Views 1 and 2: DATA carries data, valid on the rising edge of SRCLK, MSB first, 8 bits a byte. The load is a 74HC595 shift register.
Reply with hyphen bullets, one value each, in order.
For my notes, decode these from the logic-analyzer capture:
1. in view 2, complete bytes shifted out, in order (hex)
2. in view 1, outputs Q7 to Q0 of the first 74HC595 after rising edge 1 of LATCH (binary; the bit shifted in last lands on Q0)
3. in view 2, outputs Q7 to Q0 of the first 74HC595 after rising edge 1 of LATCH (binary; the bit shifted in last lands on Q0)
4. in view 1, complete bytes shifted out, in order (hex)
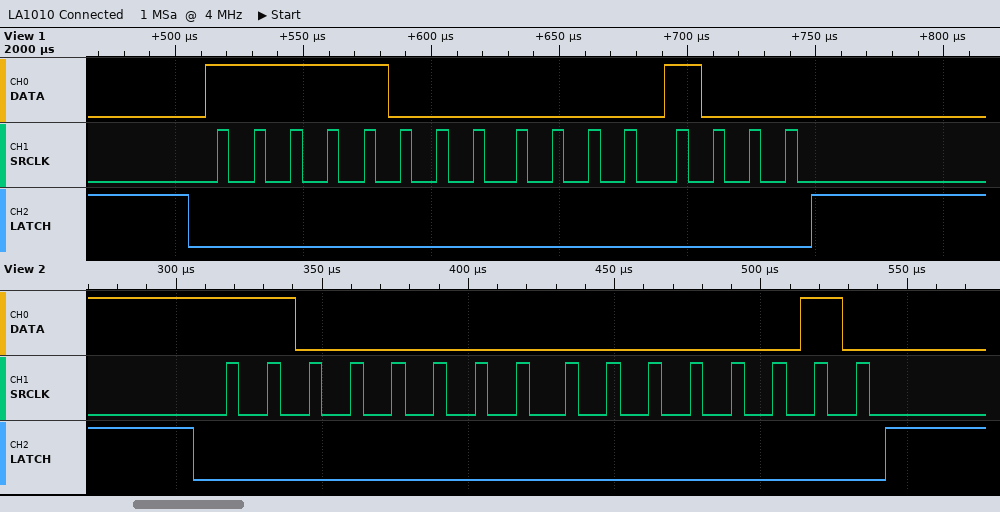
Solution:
- 0xC0 0x02
- 00001000
- 00000010
- 0xF8 0x08
